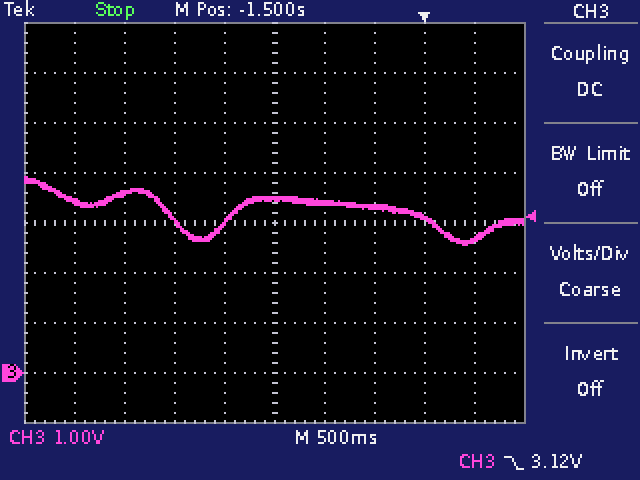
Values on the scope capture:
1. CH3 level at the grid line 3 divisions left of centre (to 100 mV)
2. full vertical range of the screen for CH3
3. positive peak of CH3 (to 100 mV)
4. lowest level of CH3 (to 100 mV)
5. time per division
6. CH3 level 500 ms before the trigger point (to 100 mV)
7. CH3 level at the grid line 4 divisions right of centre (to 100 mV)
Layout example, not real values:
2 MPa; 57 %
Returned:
3.6 V; 8 V; 3.9 V; 2.6 V; 500 ms; 3.3 V; 2.7 V
